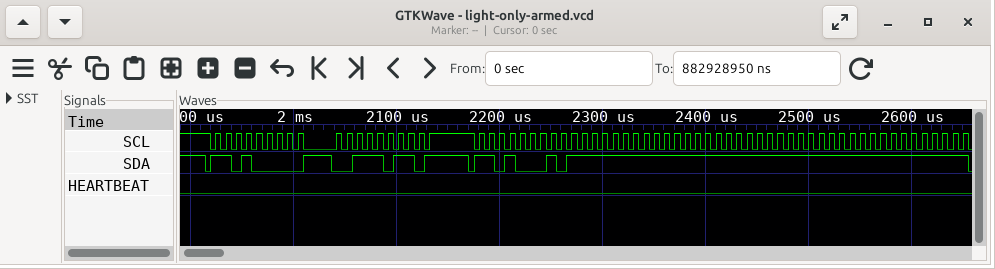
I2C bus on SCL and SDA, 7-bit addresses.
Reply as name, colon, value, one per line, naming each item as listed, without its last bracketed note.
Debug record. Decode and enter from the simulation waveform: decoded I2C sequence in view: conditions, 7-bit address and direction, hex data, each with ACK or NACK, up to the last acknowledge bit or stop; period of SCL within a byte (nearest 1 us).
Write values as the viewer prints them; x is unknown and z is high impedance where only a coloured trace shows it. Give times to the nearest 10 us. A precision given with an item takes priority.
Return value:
decoded I2C sequence in view: conditions, 7-bit address and direction, hex data, each with ACK or NACK, up to the last acknowledge bit or stop: start, address 68 write ACK, 3B ACK, repeated start, address 68 read ACK, FF NACK, FF NACK, FF NACK, FF NACK
period of SCL within a byte: 10 us
